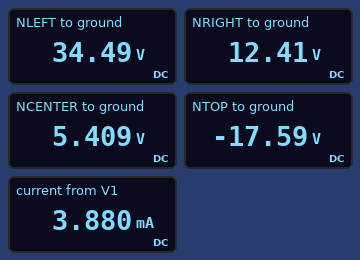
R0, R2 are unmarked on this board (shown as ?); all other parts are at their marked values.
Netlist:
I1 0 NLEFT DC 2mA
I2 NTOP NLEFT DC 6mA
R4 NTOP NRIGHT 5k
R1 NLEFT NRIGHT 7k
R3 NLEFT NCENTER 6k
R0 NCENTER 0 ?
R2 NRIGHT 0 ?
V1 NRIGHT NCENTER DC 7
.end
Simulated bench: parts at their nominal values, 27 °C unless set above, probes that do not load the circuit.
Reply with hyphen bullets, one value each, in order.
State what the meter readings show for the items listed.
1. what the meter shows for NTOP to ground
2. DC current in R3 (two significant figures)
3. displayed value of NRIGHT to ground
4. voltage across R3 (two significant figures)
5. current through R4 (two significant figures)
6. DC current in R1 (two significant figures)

- -17.59 V
- 4.8 mA
- 12.41 V
- 29 V
- 6.0 mA
- 3.2 mA
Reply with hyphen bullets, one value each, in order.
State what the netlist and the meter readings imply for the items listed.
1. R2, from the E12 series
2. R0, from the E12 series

- 12 kΩ
- 5.6 kΩ
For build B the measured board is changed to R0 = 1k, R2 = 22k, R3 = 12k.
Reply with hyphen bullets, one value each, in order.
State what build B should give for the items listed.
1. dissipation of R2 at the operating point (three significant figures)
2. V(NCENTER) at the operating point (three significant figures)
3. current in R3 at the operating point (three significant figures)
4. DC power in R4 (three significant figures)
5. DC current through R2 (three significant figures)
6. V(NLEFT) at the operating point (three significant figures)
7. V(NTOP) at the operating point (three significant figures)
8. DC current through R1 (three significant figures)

- 3.37 mW
- 1.61 V
- 3.32 mA
- 180 mW
- 391 µA
- 41.4 V
- -21.4 V
- 4.68 mA
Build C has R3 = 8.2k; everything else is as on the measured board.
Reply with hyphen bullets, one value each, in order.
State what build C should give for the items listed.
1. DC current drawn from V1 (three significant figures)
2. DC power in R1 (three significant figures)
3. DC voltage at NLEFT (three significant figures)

- 3.18 mA
- 104 mW
- 39.4 V
